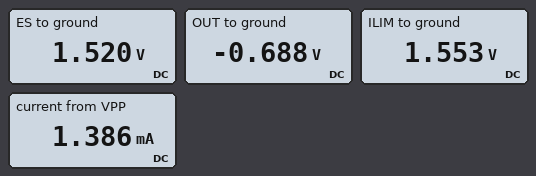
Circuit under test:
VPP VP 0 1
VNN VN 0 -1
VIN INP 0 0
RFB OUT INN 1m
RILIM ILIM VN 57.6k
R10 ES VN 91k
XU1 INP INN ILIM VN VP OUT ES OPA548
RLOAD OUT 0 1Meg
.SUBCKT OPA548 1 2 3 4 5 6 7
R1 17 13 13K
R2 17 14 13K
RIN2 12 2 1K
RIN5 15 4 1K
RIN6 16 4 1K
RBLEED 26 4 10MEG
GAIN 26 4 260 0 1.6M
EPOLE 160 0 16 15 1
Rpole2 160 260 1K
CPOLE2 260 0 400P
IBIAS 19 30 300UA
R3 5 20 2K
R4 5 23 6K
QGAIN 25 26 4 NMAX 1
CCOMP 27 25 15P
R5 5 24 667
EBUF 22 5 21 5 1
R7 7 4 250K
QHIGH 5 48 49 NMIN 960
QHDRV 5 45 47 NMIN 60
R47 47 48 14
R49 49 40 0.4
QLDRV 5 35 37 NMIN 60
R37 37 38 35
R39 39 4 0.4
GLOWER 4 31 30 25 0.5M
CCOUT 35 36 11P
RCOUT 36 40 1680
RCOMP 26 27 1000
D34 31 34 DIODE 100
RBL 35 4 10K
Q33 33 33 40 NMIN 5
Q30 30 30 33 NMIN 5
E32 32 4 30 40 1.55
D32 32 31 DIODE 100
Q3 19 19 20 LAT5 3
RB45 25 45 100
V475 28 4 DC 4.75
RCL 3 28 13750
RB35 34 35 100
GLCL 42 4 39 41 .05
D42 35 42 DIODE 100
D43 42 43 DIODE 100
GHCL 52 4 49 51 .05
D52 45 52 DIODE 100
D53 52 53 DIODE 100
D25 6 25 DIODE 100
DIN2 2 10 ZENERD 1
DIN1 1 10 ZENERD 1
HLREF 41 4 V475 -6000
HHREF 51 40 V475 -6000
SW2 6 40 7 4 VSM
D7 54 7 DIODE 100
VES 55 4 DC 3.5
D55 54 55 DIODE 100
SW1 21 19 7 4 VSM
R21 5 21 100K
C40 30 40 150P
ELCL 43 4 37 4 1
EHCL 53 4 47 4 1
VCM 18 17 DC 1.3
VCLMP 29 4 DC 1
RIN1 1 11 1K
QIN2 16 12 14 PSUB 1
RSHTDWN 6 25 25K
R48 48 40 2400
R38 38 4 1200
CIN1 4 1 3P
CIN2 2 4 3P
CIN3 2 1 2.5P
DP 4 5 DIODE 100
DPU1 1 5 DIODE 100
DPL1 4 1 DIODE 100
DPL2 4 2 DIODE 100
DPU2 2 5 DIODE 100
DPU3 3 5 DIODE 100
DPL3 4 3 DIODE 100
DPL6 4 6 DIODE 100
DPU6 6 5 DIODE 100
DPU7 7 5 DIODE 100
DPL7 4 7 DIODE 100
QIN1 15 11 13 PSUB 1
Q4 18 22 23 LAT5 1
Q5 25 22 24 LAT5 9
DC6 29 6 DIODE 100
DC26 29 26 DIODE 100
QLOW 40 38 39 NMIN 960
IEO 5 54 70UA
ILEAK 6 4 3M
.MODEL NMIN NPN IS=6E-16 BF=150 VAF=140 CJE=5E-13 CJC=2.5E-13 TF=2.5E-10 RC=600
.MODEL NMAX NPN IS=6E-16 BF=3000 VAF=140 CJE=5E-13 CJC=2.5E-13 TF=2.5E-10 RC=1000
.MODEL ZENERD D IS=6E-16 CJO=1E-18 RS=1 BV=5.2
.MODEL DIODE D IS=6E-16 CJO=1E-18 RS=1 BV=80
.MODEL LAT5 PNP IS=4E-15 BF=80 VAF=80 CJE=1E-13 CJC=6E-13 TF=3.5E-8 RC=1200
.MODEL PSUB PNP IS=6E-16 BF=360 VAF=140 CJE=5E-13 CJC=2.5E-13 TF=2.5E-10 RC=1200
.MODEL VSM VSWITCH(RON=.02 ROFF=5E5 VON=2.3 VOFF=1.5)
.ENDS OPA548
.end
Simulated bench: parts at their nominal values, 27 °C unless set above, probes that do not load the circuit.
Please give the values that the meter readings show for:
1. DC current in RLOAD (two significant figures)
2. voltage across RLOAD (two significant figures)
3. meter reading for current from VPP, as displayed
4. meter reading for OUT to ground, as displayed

690 nA
690 mV
1.386 mA
-0.688 V
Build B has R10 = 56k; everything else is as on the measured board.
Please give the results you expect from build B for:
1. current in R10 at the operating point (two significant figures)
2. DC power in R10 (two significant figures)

45 µA
110 µW
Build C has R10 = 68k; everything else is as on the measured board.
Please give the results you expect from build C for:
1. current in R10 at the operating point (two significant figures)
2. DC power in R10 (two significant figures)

37 µA
93 µW
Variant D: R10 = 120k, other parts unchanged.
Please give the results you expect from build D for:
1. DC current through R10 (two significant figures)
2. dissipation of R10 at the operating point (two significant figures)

21 µA
53 µW
